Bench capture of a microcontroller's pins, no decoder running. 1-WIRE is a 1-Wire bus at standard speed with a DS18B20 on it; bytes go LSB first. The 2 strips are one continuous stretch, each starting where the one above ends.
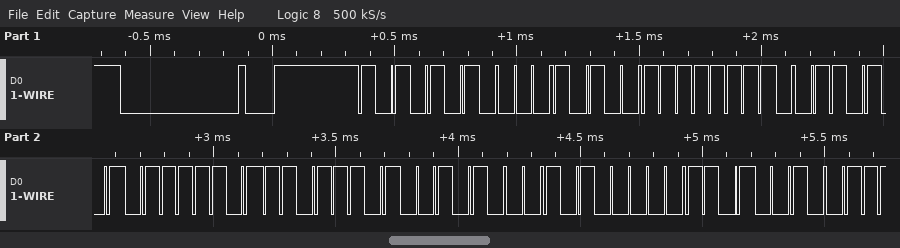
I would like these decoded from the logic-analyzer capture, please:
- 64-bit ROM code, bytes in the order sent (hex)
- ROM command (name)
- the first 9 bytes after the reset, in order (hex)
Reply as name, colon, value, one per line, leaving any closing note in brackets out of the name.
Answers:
64-bit ROM code, bytes in the order sent: 28 FF AC BE BB 14 05 4B
ROM command: Match ROM
the first 9 bytes after the reset, in order: 55 28 FF AC BE BB 14 05 4B
